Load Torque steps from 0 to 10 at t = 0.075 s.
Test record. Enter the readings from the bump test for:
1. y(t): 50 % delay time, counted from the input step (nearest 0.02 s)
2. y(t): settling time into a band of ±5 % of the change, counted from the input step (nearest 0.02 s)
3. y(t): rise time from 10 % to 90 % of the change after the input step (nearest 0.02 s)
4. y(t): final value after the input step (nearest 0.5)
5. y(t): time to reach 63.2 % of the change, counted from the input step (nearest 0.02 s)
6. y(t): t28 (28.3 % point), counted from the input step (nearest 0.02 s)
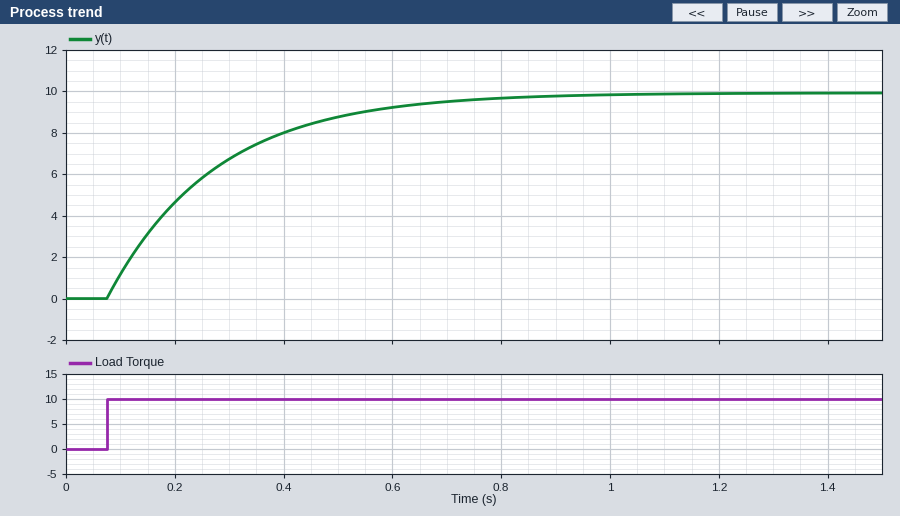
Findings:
0.14 s
0.60 s
0.44 s
10.0
0.20 s
0.06 s
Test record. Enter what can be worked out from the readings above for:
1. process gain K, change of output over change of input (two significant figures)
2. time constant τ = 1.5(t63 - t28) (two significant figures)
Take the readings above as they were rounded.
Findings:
1.0
0.21 s
